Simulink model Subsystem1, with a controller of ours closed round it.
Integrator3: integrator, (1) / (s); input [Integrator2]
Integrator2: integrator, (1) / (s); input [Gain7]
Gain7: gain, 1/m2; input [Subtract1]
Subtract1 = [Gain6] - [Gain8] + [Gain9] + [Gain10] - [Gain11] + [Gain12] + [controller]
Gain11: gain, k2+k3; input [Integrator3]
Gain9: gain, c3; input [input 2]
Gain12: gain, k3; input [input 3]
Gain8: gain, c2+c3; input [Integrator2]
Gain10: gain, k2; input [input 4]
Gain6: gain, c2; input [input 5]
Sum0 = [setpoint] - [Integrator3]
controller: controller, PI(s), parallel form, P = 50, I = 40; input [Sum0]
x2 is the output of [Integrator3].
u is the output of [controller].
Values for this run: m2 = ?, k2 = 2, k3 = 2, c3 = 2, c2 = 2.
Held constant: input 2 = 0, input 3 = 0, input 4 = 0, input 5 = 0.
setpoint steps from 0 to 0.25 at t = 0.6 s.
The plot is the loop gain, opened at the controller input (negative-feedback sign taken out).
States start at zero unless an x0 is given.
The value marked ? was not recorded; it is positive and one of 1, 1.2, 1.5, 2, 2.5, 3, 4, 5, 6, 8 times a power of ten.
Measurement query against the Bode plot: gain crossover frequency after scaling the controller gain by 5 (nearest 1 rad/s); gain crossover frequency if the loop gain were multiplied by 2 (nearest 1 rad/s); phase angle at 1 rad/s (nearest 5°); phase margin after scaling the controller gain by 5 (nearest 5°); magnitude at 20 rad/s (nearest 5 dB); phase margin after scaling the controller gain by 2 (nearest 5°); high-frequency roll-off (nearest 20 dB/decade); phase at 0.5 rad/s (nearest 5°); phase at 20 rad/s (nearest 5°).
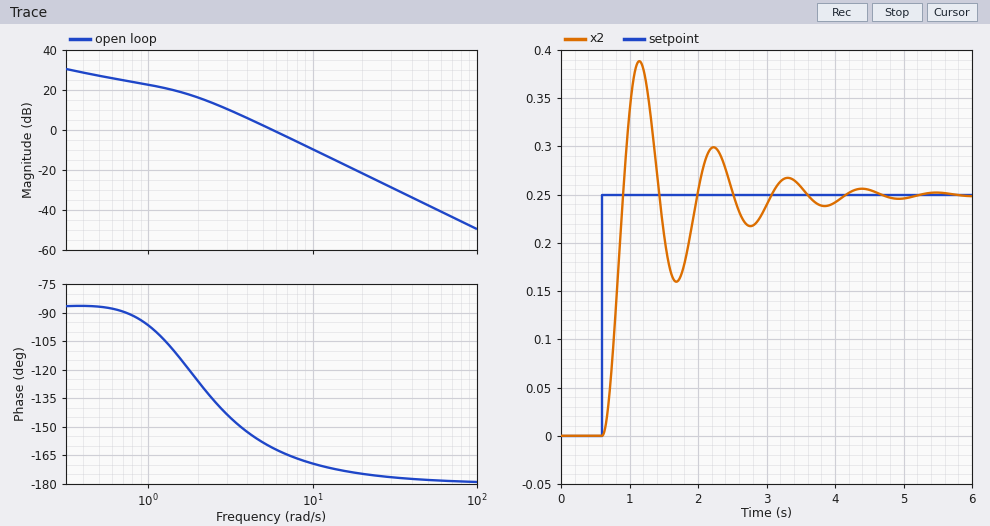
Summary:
13 rad/s
8 rad/s
-95°
10°
-20 dB
15°
-40 dB/decade
-85°
-175°
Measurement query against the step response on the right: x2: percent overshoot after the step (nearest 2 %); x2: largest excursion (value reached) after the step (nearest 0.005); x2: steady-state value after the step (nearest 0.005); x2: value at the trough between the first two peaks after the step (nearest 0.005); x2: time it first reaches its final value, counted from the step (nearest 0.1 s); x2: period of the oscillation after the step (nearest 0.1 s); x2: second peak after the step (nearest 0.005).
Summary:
56 %
0.390
0.250
0.160
0.3 s
1.1 s
0.300
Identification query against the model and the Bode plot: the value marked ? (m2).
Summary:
1.5
